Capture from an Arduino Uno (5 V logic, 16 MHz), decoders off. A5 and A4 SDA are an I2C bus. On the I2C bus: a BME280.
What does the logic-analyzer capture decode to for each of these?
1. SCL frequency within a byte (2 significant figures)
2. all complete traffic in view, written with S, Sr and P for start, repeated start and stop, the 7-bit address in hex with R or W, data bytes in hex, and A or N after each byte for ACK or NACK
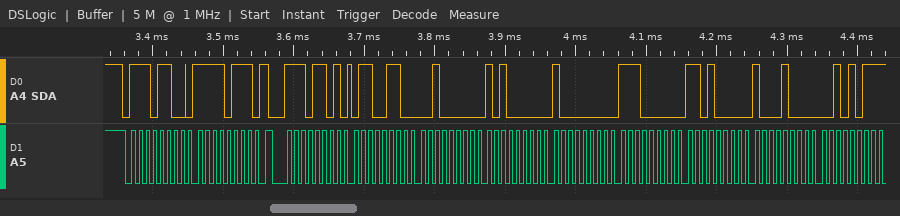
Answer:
100 kHz
S 76W A F7 A Sr 76R A 66 A 20 A A0 A 80 A E0 A D0 A 88 A 2B N
